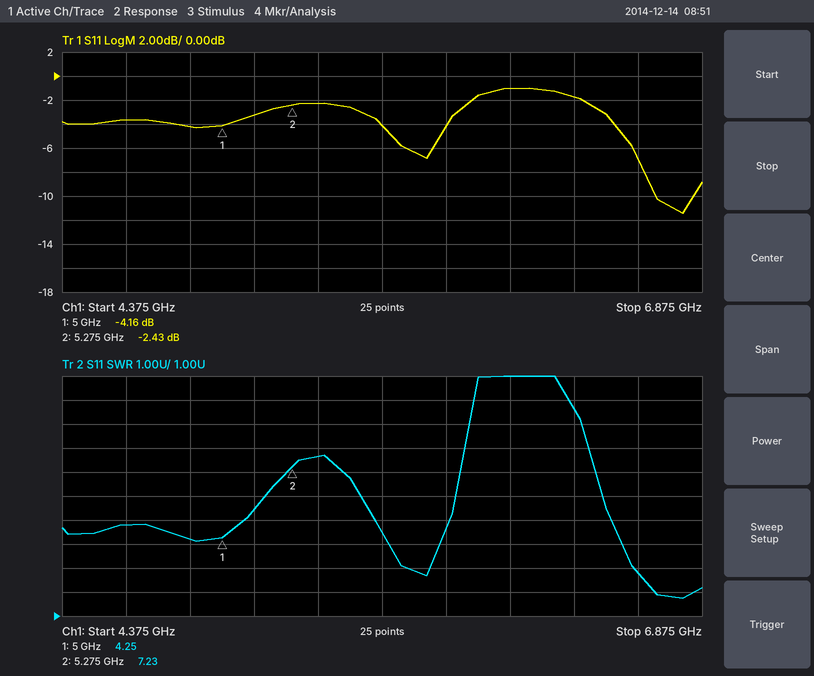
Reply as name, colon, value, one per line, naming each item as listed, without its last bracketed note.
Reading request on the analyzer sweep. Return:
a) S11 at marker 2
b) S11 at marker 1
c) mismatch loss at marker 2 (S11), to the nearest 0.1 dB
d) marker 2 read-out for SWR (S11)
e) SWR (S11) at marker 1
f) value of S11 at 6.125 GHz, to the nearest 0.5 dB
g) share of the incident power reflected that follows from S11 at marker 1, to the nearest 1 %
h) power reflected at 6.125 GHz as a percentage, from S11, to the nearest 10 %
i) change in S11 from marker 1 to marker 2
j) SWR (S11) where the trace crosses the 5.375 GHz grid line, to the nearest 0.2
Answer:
S11 at marker 2: -2.43 dB
S11 at marker 1: -4.16 dB
mismatch loss at marker 2 (S11), to the nearest 0.1 dB: 3.7 dB
marker 2 read-out for SWR: 7.23
SWR (S11) at marker 1: 4.25
value of S11 at 6.125 GHz, to the nearest 0.5 dB: -1.0 dB
share of the incident power reflected that follows from S11 at marker 1, to the nearest 1 %: 38 %
power reflected at 6.125 GHz as a percentage, from S11, to the nearest 10 %: 80 %
change in S11 from marker 1 to marker 2: 1.73 dB
SWR (S11) where the trace crosses the 5.375 GHz grid line, to the nearest 0.2: 7.6
